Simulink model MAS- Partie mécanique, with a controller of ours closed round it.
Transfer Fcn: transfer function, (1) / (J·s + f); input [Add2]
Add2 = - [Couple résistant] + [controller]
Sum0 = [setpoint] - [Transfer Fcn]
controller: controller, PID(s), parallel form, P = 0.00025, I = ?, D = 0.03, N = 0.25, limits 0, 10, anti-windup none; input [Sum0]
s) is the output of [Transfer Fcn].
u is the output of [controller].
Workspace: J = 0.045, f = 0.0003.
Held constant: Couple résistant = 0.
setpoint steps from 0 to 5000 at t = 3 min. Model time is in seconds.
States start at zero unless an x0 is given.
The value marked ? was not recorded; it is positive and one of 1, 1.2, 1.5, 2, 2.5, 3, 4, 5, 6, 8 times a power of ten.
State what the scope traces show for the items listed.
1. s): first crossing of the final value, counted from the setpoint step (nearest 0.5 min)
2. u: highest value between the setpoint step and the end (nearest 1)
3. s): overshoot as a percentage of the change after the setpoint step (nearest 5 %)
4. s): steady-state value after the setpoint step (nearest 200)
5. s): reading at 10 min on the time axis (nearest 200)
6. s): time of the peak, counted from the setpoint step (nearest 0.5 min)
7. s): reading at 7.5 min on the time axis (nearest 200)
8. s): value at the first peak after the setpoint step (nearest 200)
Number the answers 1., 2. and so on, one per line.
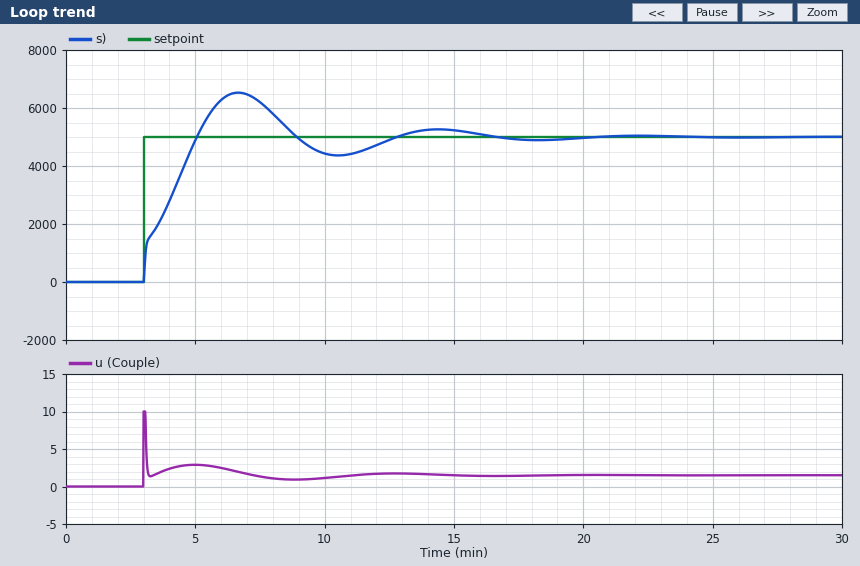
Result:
1. 2.0 min
2. 10
3. 30 %
4. 5000
5. 4400
6. 3.5 min
7. 6200
8. 6600
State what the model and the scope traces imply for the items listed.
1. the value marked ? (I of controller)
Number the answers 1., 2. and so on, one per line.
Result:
1. 1.5e-05
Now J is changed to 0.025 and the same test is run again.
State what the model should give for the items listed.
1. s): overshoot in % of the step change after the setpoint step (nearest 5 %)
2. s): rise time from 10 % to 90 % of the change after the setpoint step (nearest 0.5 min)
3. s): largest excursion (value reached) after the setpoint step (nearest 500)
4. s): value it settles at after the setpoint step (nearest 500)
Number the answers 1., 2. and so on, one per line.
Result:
1. 20 %
2. 1.5 min
3. 6000
4. 5000
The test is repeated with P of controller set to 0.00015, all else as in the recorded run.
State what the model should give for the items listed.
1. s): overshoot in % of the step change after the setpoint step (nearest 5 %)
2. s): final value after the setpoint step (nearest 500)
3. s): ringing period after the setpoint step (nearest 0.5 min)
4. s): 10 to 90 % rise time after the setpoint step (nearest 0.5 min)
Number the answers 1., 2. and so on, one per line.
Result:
1. 35 %
2. 5000
3. 7.5 min
4. 2.0 min
